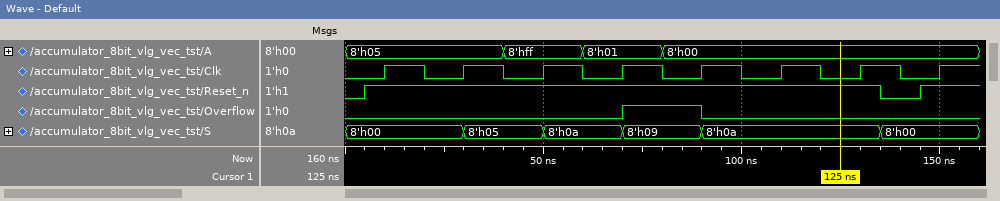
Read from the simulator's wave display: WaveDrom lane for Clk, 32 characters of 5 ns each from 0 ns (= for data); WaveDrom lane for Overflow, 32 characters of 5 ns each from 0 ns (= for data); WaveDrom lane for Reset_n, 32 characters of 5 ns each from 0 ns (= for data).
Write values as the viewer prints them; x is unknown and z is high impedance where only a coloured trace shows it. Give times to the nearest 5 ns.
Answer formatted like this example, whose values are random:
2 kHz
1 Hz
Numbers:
{name: 'Clk', wave: '0.1.0.1.0.1.0.1.0.1.0.1.0.1.0.1.'}
{name: 'Overflow', wave: '0.............1...0.............'}
{name: 'Reset_n', wave: '01.........................0.1..'}
